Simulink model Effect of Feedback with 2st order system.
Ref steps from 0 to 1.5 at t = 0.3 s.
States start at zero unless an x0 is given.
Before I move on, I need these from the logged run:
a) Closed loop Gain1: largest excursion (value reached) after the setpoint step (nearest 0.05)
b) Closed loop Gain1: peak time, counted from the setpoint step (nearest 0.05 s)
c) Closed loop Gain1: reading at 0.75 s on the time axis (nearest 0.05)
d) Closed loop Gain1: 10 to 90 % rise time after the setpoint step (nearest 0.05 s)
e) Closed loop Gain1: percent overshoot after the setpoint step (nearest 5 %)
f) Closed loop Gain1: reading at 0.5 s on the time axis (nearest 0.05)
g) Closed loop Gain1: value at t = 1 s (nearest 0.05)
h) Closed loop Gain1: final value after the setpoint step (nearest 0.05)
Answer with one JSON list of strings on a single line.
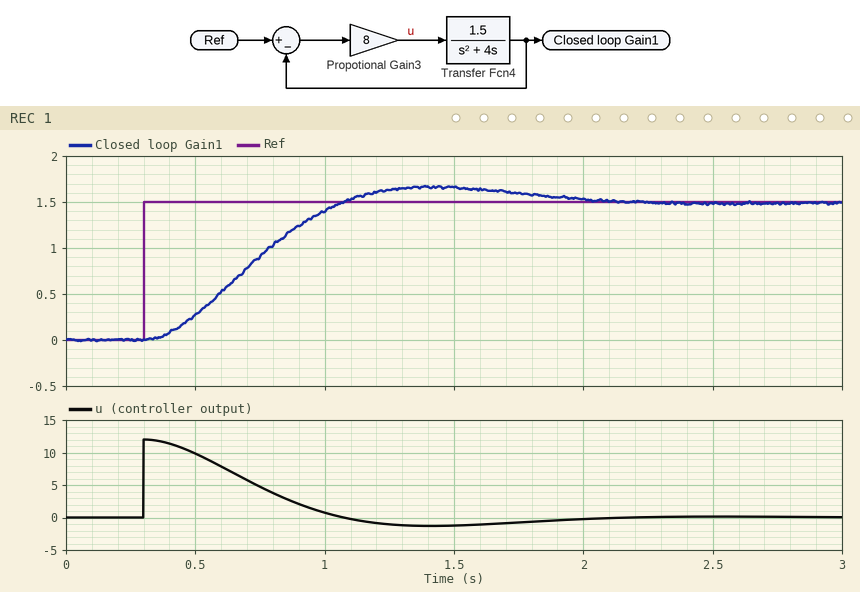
["1.65", "1.10 s", "0.90", "0.50 s", "10 %", "0.25", "1.40", "1.50"]
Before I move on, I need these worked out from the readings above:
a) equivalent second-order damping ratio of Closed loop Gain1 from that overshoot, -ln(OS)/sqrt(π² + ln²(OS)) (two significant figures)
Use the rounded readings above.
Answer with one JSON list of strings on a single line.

["0.59"]
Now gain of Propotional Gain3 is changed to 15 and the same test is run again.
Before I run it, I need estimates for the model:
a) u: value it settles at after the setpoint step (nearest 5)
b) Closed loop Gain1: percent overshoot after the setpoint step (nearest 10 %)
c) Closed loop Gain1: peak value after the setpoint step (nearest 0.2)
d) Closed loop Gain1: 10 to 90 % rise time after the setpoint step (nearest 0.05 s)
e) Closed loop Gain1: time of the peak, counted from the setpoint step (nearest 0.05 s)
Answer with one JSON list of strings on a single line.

["0", "20 %", "1.8", "0.30 s", "0.75 s"]
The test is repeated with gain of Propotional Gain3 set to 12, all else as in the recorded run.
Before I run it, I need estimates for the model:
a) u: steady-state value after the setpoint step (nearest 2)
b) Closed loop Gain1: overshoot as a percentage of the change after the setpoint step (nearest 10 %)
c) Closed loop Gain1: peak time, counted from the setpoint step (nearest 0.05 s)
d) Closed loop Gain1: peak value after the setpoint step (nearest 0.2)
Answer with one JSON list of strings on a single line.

["0", "20 %", "0.85 s", "1.8"]
